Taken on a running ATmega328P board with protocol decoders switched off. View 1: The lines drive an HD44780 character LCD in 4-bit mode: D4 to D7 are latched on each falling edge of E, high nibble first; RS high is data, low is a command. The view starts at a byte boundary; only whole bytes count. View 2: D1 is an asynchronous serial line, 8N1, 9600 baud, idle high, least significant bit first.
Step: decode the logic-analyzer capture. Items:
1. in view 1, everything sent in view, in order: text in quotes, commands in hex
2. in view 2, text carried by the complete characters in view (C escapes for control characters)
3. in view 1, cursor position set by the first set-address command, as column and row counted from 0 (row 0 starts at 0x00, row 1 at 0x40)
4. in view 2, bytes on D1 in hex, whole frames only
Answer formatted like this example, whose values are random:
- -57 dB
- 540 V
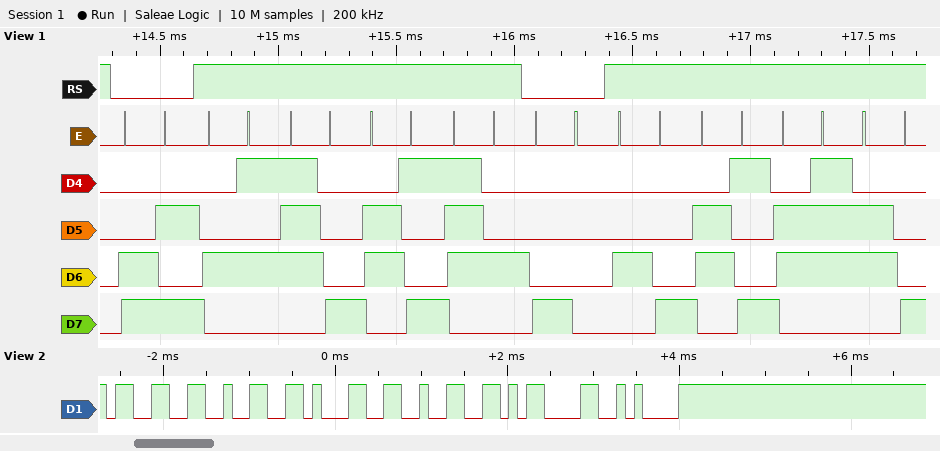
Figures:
- 0xCA "Exit" 0x80 "High"
- "3212\r\n"
- column 10, row 1
- 33 32 31 32 0D 0A
